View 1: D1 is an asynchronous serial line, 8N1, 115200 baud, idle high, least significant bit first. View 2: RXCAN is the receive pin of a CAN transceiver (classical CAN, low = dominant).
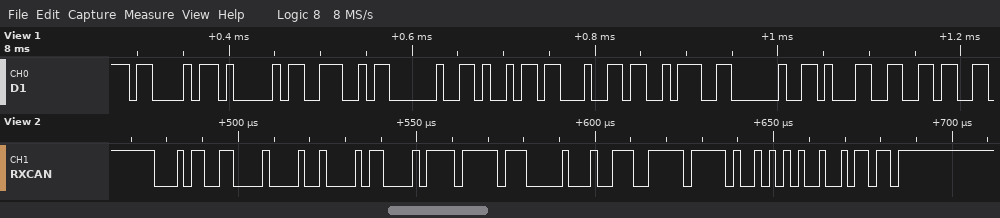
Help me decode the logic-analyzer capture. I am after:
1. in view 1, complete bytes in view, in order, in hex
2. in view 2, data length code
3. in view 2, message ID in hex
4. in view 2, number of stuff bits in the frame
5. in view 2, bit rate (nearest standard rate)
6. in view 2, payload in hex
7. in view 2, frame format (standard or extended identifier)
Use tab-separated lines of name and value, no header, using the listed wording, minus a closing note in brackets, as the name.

in view 1, complete bytes in view, in order, in hex	43 41 4E 20 69 64 3A 20 31 36
in view 2, data length code	8
in view 2, message ID in hex	0x166
in view 2, number of stuff bits in the frame	4
in view 2, bit rate	500 kbit/s
in view 2, payload in hex	48 58 5E FF 00 9C FF E5
in view 2, frame format	standard
